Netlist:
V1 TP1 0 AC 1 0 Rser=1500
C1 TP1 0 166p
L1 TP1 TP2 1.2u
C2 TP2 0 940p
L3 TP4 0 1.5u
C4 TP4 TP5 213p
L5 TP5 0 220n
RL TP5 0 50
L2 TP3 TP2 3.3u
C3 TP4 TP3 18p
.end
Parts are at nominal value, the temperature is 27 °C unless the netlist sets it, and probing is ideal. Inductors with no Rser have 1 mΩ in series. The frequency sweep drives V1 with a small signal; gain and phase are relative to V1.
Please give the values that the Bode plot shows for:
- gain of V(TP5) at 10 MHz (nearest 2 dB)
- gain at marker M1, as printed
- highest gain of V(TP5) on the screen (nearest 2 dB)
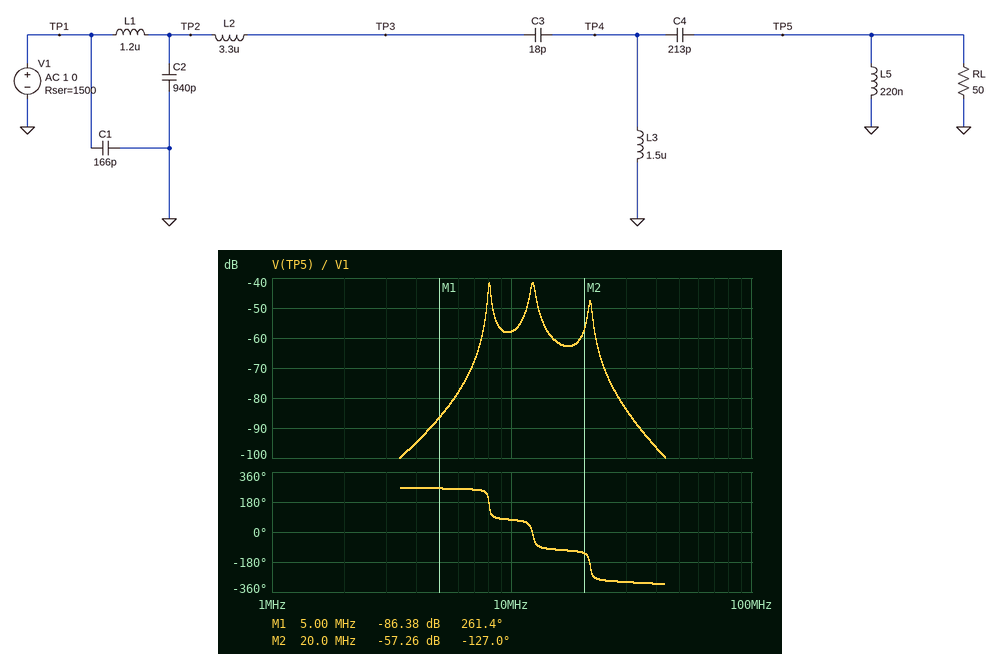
-58 dB
-86.38 dB
-42 dB
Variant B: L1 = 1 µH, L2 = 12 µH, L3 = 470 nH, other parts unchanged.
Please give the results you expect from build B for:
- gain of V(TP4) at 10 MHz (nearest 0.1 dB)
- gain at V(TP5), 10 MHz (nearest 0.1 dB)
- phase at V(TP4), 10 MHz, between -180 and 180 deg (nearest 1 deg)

-36.9 dB
-50.3 dB
81 deg
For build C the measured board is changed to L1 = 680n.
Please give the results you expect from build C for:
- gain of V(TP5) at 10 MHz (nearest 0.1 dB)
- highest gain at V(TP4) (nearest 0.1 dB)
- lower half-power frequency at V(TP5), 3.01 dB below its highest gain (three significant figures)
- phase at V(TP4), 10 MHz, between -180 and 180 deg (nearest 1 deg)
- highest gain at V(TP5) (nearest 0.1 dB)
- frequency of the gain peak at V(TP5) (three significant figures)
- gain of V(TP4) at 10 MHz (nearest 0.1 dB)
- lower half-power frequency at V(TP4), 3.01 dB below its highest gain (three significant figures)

-63.3 dB
-26.4 dB
15.9 MHz
-84 deg
-35.3 dB
16.2 MHz
-49.9 dB
7.95 MHz
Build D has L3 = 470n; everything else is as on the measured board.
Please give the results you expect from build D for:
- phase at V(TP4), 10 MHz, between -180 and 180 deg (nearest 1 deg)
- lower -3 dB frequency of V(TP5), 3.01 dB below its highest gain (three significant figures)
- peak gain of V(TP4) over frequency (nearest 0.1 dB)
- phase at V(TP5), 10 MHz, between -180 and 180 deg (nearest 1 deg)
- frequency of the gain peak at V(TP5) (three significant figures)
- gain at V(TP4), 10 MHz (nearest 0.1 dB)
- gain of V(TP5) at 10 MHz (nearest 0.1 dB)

81 deg
12.0 MHz
-22.6 dB
-118 deg
12.3 MHz
-51.8 dB
-65.2 dB
